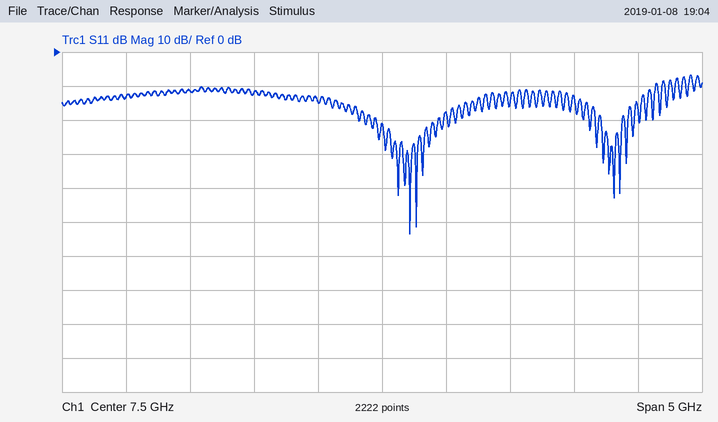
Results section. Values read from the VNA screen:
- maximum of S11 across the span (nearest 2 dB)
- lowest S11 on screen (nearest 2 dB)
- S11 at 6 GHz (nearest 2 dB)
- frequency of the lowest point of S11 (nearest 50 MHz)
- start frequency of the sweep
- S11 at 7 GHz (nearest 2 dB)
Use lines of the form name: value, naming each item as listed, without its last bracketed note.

maximum of S11 across the span: -6 dB
lowest S11 on screen: -54 dB
S11 at 6 GHz: -12 dB
frequency of the lowest point of S11: 7.70 GHz
start frequency of the sweep: 5 GHz
S11 at 7 GHz: -14 dB
